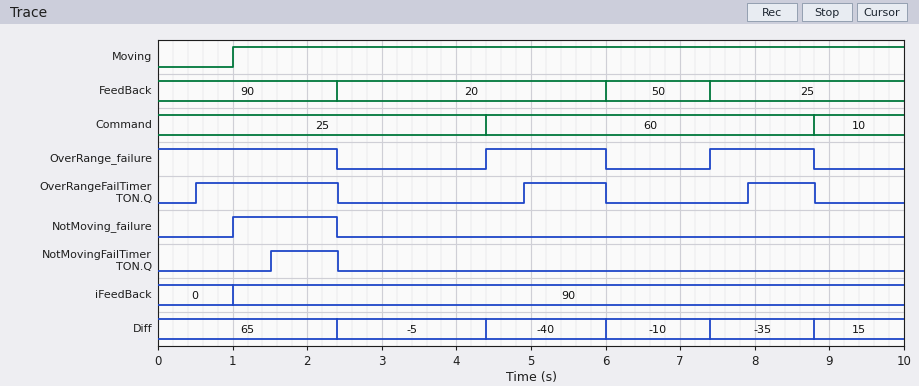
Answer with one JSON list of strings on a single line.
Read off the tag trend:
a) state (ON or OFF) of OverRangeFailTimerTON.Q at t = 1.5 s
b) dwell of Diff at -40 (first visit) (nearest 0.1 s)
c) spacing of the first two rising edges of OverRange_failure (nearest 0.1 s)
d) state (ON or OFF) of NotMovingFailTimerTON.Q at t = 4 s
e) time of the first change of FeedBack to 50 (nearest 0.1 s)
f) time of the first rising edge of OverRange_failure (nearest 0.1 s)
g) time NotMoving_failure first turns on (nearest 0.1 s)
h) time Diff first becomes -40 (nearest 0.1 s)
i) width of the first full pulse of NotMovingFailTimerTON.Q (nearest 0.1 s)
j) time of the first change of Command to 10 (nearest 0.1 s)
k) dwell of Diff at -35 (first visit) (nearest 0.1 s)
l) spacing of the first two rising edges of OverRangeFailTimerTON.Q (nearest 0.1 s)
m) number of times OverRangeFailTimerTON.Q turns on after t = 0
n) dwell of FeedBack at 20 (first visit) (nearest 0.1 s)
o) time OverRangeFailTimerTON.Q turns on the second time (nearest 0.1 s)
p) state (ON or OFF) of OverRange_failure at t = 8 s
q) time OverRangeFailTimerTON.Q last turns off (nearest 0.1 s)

["ON", "1.6 s", "3.0 s", "OFF", "6.0 s", "4.4 s", "1.0 s", "4.4 s", "0.9 s", "8.8 s", "1.4 s", "4.4 s", "3", "3.6 s", "4.9 s", "ON", "8.8 s"]
